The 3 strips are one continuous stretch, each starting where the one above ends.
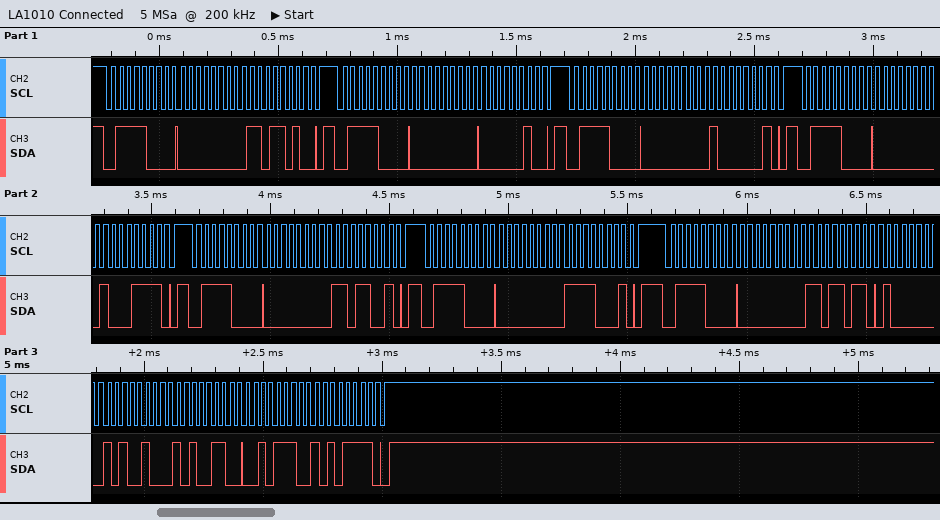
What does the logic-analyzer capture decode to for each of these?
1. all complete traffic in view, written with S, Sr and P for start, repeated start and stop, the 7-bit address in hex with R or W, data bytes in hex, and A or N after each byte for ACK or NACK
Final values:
S 3CW A 00 A DA A P S 3CW A 00 A 02 A P S 3CW A 00 A 81 A P S 3CW A 00 A 8F A P S 3CW A 00 A D9 A P S 3CW A 00 A F1 A P S 3CW A 00 A DB A 40 A A4 A A6 A 2E A AF A P
